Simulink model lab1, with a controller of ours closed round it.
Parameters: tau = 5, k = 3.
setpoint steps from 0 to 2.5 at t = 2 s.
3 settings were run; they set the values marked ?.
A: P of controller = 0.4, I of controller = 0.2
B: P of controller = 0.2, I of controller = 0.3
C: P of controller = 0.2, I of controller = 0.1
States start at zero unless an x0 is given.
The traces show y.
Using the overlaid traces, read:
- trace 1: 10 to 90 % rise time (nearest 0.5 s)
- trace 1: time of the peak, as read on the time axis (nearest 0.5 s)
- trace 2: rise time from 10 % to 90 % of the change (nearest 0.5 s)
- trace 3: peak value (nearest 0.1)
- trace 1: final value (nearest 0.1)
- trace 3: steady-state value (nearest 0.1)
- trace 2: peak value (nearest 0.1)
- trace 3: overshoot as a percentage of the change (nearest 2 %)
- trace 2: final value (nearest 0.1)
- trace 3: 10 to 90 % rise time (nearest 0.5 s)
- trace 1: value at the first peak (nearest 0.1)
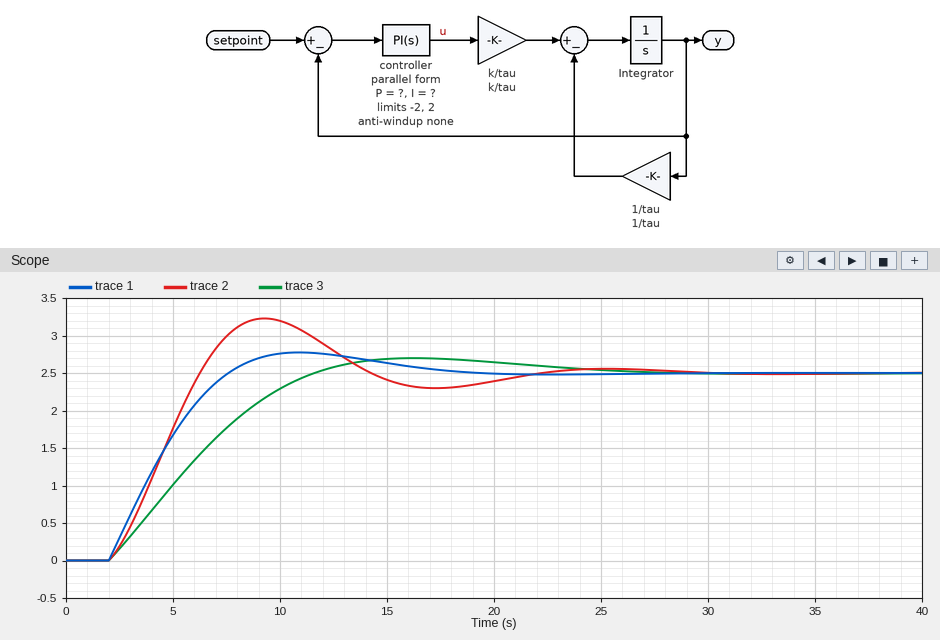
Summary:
4.0 s
11.0 s
3.0 s
2.7
2.5
2.5
3.2
8 %
2.5
7.0 s
2.8
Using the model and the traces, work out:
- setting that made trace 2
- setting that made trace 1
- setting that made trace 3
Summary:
B
A
C
